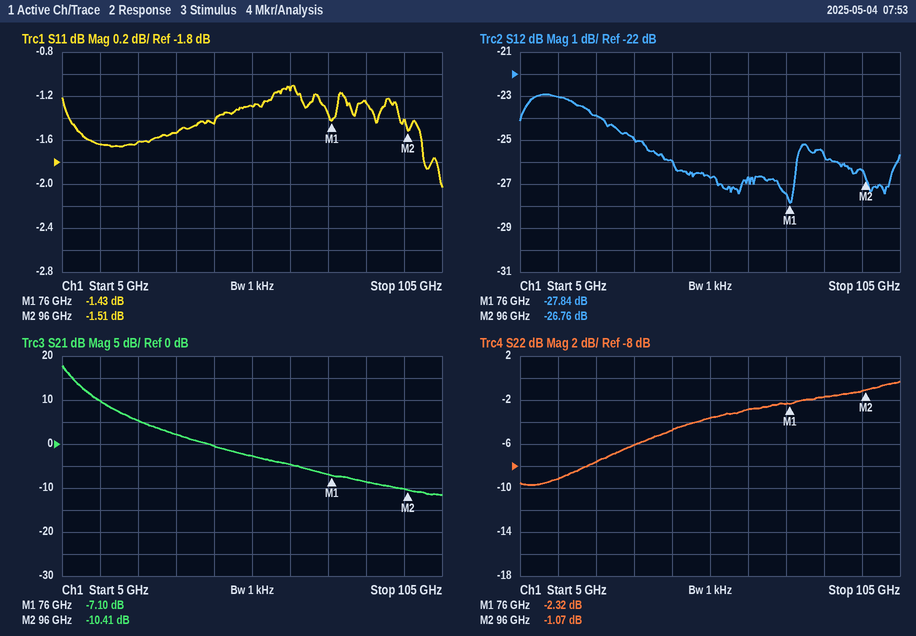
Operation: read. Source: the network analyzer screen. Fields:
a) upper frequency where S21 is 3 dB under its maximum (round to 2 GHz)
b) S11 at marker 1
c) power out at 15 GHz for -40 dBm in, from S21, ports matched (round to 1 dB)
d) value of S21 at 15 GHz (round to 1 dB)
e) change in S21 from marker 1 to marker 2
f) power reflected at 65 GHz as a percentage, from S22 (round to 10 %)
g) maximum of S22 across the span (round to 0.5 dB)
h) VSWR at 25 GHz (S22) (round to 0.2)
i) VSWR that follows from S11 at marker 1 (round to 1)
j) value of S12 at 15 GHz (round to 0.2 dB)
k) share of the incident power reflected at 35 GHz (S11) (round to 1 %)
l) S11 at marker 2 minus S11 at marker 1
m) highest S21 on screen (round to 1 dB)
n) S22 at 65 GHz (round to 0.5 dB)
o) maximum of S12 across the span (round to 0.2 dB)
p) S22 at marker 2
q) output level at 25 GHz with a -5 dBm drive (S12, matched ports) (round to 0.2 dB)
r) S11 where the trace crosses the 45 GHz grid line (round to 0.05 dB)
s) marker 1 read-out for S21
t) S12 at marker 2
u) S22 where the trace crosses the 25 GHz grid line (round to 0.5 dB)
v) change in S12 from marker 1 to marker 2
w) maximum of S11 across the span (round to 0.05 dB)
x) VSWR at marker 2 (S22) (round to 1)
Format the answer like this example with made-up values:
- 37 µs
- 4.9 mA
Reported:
- 8 GHz
- -1.43 dB
- -30 dBm
- 10 dB
- -3.31 dB
- 50 %
- -0.5 dB
- 2.4
- 12
- -23.0 dB
- 70 %
- -0.08 dB
- 18 dB
- -3.0 dB
- -23.0 dB
- -1.07 dB
- -28.8 dBm
- -1.45 dB
- -7.10 dB
- -26.76 dB
- -7.5 dB
- 1.08 dB
- -1.10 dB
- 16
